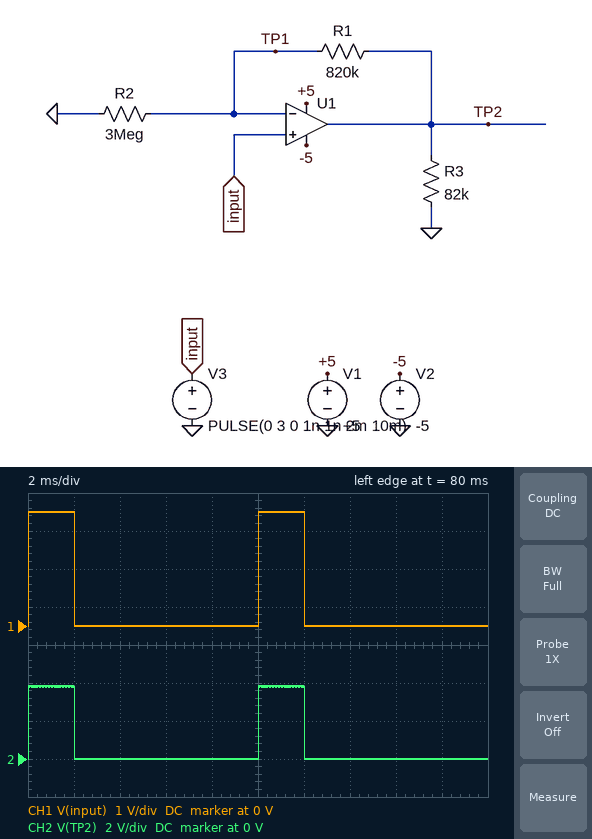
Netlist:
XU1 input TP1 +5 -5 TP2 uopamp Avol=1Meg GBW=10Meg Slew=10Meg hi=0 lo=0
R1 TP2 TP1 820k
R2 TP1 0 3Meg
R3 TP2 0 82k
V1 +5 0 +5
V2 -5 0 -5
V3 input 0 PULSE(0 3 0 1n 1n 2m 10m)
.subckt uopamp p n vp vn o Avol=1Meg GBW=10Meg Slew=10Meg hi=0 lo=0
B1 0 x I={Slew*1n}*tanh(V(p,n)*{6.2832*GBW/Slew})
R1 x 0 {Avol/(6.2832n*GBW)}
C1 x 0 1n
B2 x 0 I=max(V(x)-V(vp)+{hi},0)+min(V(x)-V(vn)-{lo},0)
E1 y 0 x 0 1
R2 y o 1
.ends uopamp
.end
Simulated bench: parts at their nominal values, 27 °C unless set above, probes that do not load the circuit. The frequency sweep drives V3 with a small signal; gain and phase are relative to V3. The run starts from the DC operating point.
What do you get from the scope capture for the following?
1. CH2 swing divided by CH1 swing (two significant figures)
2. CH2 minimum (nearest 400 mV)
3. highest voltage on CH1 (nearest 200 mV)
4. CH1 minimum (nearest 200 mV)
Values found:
1.3
0 V
3.0 V
0 V
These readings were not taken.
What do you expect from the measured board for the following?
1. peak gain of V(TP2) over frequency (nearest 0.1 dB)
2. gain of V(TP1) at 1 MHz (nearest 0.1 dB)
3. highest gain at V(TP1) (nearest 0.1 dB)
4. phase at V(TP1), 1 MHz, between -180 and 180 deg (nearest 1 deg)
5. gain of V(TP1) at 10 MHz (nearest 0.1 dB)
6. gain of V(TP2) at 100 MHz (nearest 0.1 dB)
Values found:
2.1 dB
-0.1 dB
0 dB
-7 deg
-4.2 dB
-20.0 dB
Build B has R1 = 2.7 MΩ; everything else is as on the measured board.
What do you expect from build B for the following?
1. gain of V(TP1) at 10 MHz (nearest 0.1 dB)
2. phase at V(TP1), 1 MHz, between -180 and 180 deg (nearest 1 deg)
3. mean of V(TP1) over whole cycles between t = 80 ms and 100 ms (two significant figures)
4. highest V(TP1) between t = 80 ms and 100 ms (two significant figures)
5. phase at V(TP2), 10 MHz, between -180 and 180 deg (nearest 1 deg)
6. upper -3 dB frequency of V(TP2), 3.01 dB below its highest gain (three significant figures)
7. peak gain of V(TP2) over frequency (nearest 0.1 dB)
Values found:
-6.6 dB
-11 deg
530 mV
2.6 V
-62 deg
5.26 MHz
5.6 dB
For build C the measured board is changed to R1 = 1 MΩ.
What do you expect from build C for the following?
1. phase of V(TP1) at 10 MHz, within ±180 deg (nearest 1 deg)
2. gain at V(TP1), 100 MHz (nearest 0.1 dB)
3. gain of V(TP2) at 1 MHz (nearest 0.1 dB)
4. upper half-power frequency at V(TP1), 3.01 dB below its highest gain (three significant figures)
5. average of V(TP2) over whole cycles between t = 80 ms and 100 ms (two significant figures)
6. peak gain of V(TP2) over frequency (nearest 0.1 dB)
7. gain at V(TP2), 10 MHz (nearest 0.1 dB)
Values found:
-53 deg
-22.5 dB
2.4 dB
7.50 MHz
800 mV
2.5 dB
-1.9 dB
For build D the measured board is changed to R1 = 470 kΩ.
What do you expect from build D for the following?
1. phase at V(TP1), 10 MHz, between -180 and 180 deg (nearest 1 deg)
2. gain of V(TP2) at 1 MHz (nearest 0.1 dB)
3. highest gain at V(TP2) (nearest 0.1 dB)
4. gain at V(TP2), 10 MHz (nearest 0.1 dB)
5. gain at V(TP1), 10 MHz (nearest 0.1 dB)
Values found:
-49 deg
1.2 dB
1.3 dB
-2.4 dB
-3.7 dB
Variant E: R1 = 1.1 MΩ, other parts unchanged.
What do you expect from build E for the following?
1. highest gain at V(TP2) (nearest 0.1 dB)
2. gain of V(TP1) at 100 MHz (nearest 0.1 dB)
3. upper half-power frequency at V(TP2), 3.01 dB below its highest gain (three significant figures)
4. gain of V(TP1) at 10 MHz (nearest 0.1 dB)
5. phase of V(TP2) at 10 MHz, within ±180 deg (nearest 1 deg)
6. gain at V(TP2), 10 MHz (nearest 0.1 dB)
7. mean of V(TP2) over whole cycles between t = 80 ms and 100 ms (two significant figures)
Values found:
2.7 dB
-22.7 dB
7.32 MHz
-4.6 dB
-54 deg
-1.9 dB
820 mV
